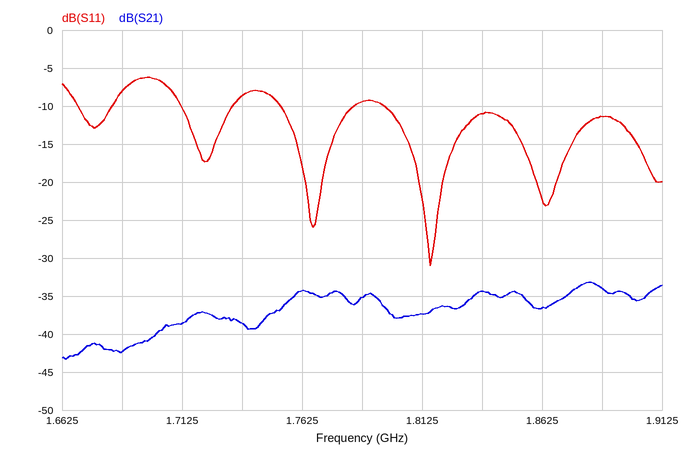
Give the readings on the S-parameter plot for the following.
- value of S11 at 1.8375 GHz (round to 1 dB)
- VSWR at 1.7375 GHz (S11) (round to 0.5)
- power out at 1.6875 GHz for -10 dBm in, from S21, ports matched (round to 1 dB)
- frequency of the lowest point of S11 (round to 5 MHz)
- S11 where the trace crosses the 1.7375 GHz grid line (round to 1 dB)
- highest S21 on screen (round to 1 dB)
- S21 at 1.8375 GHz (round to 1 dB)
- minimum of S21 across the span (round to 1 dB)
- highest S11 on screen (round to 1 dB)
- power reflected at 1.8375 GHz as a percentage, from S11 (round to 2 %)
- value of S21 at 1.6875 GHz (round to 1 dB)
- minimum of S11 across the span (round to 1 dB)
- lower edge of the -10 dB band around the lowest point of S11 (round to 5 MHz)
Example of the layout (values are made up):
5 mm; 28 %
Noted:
-11 dB; 2.0; -52 dBm; 1.815 GHz; -9 dB; -33 dB; -34 dB; -43 dB; -6 dB; 8 %; -42 dB; -31 dB; 1.795 GHz
